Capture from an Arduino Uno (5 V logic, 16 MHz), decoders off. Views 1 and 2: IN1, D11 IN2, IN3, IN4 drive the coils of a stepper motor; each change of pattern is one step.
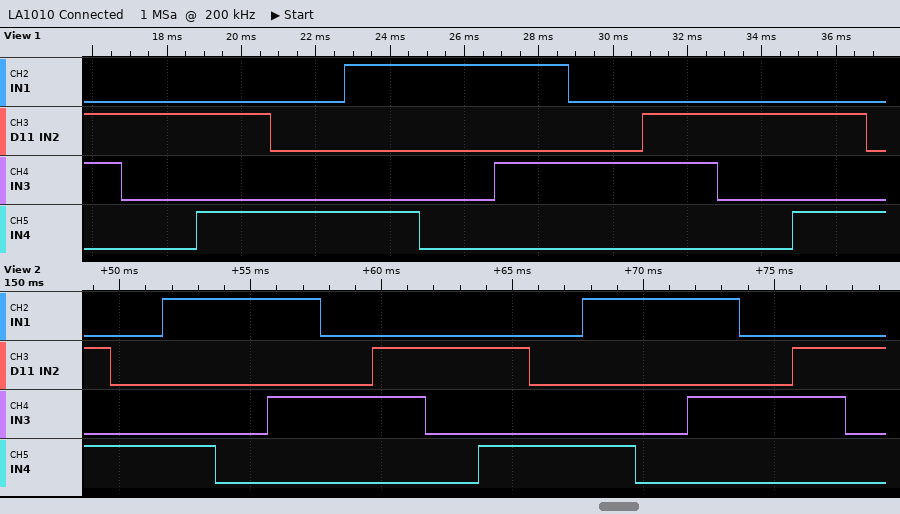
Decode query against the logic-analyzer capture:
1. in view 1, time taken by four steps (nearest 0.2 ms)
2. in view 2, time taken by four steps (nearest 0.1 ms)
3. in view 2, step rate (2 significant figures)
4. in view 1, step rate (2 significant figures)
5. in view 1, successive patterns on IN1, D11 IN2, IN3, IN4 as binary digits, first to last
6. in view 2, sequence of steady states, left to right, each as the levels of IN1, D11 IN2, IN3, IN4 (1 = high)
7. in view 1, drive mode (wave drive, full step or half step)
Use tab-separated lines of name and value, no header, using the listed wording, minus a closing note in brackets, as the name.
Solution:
in view 1, time taken by four steps	8.0 ms
in view 2, time taken by four steps	8.0 ms
in view 2, step rate	500 steps/s
in view 1, step rate	500 steps/s
in view 1, successive patterns on IN1, D11 IN2, IN3, IN4 as binary digits, first to last	0110 0100 0101 0001 1001 1000 1010 0010 0110 0100 0101 0001
in view 2, sequence of steady states, left to right, each as the levels of IN1, D11 IN2, IN3, IN4	0101 0001 1001 1000 1010 0010 0110 0100 0101 0001 1001 1000 1010 0010 0110 0100
in view 1, drive mode	half step
